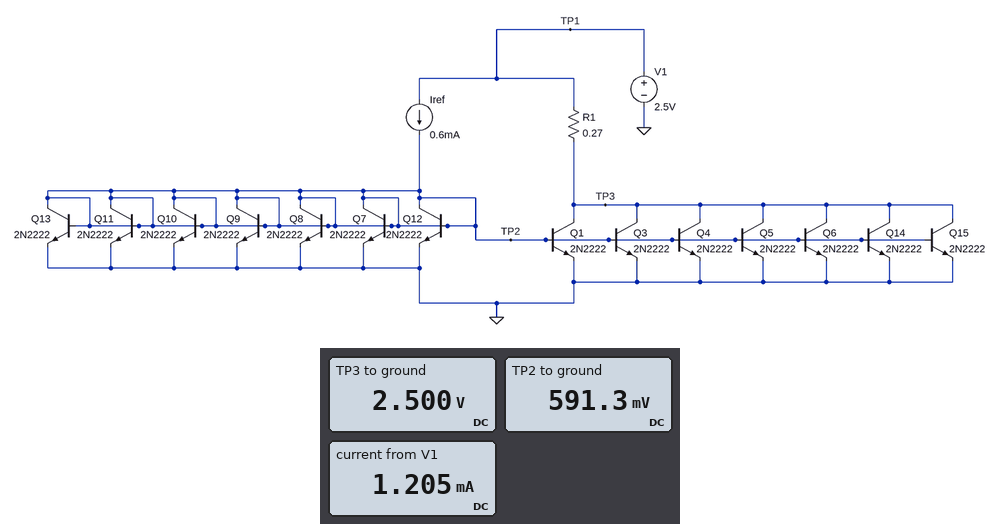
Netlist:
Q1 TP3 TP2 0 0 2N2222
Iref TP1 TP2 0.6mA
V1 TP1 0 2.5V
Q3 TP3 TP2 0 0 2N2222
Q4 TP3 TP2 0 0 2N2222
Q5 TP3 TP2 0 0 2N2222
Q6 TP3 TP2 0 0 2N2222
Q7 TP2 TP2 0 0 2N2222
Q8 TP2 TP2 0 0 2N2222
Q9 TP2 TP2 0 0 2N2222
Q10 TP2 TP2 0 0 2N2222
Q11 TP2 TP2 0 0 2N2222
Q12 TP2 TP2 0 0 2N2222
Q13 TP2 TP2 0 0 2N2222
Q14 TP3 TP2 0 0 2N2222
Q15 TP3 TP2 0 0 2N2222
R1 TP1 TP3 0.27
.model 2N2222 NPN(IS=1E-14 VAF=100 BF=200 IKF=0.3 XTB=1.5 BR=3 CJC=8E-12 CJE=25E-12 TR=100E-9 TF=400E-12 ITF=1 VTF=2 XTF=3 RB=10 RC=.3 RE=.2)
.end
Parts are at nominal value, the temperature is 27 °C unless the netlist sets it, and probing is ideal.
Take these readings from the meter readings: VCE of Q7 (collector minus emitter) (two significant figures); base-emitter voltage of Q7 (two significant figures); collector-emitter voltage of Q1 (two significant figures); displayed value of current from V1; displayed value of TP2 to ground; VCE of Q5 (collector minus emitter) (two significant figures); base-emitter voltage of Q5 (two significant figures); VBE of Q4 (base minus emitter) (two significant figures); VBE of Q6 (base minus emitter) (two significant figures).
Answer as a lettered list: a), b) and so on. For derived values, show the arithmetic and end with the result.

a) 591.3 mV = 590 mV
b) 591.3 mV = 590 mV
c) 2.5 V = 2.5 V
d) 1.205 mA
e) 591.3 mV
f) 2.5 V = 2.5 V
g) 591.3 mV = 590 mV
h) 591.3 mV = 590 mV
i) 591.3 mV = 590 mV
